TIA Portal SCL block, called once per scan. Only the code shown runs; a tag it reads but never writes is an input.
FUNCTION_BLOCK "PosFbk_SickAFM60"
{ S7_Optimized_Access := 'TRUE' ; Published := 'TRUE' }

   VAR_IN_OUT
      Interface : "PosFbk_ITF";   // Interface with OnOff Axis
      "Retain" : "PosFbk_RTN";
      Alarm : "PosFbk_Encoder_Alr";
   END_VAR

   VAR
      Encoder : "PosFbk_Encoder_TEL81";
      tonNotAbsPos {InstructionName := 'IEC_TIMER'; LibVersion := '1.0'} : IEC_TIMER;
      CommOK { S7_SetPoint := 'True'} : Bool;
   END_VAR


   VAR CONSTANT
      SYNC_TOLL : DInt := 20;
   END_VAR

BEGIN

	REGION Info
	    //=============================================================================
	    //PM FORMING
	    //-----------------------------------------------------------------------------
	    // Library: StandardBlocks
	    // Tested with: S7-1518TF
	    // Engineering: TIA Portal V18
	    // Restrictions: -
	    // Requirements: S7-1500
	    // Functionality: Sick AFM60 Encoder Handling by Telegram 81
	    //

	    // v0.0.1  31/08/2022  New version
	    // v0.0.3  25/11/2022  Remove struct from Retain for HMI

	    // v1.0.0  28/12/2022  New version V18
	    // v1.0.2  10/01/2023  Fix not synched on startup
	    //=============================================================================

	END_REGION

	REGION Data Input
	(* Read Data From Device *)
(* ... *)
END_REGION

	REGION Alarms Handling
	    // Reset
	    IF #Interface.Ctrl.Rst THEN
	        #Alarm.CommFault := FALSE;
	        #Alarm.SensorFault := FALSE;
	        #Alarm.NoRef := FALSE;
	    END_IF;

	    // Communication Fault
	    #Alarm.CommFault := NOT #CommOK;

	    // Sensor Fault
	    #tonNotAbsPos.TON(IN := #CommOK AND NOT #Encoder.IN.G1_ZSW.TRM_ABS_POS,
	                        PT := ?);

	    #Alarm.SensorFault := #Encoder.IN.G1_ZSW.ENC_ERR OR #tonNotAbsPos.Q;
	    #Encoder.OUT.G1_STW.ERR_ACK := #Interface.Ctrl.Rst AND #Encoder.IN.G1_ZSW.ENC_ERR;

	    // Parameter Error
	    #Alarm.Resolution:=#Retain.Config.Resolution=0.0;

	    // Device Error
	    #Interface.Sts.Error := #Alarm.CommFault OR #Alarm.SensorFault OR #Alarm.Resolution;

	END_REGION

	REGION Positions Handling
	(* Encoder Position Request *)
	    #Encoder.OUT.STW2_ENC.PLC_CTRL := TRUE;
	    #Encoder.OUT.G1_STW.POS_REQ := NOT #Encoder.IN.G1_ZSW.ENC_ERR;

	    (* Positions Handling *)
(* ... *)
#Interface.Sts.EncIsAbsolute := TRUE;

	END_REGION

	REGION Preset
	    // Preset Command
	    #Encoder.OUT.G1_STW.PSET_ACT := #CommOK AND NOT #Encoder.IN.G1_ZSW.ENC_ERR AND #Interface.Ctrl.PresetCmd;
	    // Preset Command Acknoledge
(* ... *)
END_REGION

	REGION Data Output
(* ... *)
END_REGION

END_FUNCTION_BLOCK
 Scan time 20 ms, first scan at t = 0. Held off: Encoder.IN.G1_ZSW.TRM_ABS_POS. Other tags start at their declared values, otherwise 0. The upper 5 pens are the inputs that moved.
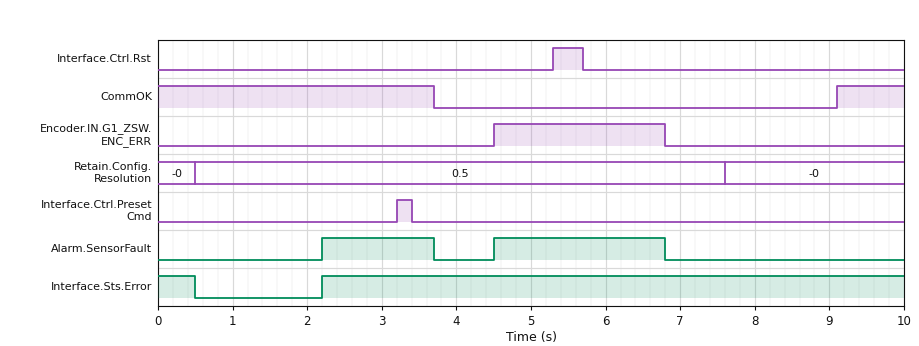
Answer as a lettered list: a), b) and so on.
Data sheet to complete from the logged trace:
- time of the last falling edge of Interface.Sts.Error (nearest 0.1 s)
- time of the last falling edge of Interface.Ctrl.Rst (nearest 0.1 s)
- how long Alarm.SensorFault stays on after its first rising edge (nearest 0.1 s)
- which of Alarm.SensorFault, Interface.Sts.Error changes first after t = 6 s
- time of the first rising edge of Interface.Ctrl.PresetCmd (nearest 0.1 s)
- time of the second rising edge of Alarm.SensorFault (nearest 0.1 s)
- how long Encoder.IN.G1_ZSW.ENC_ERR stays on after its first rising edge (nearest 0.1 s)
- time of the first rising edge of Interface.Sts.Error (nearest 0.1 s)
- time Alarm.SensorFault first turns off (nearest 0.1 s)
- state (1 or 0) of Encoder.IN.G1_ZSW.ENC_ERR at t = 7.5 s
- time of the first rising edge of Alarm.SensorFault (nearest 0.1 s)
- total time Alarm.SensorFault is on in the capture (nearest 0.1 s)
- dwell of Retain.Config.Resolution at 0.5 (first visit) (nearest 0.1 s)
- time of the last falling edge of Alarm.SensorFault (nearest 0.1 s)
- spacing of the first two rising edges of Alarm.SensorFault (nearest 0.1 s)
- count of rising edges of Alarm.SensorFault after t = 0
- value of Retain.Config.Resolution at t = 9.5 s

a) 0.5 s
b) 5.7 s
c) 1.5 s
d) Alarm.SensorFault
e) 3.2 s
f) 4.5 s
g) 2.3 s
h) 2.2 s
i) 3.7 s
j) 0
k) 2.2 s
l) 3.8 s
m) 7.1 s
n) 6.8 s
o) 2.3 s
p) 2
q) -0
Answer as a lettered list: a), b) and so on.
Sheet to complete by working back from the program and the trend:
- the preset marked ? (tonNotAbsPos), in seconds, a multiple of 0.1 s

a) 2.2 s
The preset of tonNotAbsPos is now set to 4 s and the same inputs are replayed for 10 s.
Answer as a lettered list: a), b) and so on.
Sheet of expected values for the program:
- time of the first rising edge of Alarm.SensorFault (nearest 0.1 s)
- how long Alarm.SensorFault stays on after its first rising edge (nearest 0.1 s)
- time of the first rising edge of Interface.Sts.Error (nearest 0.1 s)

a) 4.5 s
b) 2.3 s
c) 3.7 s
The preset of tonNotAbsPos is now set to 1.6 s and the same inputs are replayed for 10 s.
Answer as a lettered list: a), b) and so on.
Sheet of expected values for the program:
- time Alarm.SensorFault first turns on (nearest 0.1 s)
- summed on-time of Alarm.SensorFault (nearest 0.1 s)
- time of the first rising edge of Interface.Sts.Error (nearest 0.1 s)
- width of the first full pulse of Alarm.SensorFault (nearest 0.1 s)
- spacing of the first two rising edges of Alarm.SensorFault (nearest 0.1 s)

a) 1.6 s
b) 4.4 s
c) 1.6 s
d) 2.1 s
e) 2.9 s
